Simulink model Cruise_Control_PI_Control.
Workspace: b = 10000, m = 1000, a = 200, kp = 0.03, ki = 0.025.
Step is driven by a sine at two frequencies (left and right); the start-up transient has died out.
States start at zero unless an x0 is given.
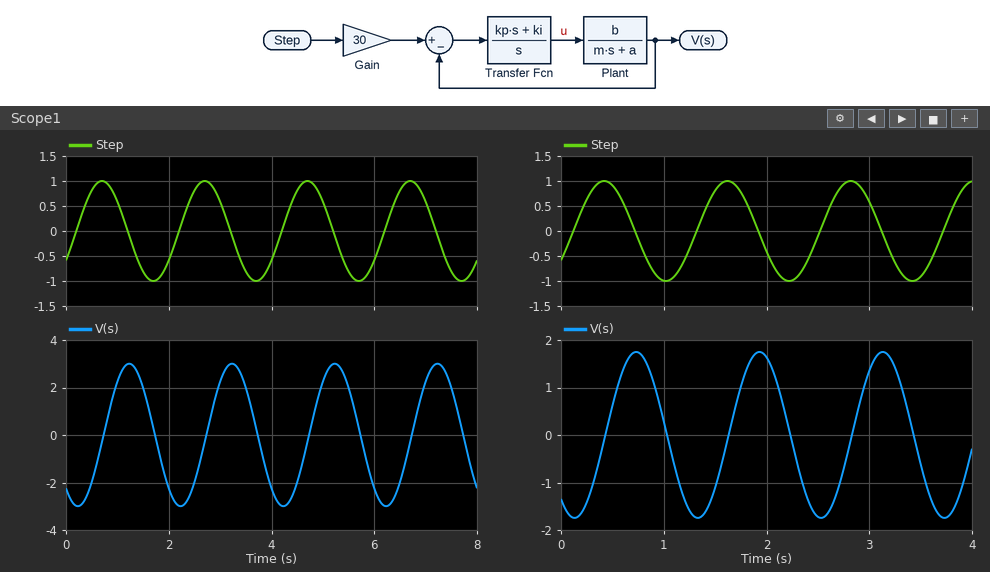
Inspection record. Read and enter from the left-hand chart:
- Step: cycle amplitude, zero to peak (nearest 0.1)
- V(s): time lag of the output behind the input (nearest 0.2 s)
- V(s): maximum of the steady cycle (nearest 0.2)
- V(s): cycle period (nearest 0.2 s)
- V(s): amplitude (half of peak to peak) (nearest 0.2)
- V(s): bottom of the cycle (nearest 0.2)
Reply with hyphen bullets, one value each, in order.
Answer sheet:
- 1.0
- 0.6 s
- 3.0
- 2.0 s
- 3.0
- -3.0
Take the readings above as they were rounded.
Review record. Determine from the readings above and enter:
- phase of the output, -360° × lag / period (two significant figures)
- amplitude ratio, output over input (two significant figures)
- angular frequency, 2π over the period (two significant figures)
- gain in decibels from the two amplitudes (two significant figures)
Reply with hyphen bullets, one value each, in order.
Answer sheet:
- -110°
- 3.0
- 3.1 rad/s
- 9.5 dB
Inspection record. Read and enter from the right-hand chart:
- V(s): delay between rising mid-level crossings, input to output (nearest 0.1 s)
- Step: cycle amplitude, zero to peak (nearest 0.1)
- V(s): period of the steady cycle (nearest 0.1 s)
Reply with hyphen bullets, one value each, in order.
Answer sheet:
- 0.3 s
- 1.0
- 1.2 s
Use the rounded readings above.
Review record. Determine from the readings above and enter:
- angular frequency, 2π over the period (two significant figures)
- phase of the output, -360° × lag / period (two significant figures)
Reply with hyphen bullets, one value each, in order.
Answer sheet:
- 5.2 rad/s
- -90°
